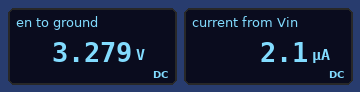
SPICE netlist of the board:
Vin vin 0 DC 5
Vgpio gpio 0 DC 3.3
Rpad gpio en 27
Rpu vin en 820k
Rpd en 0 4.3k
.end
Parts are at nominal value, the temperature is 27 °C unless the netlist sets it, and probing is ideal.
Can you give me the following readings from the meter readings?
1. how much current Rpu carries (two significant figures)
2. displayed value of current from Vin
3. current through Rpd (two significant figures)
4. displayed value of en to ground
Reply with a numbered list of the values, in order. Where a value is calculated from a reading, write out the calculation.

1. (5 V - 3.279 V) / 820 kΩ = 2.1 µA
2. 2.1 µA
3. (3.279 V) / 4.3 kΩ = 760 µA
4. 3.279 V
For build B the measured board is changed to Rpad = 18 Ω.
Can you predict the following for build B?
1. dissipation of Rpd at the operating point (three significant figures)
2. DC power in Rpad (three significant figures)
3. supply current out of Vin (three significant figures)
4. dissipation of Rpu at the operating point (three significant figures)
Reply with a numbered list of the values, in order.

1. 2.51 mW
2. 10.5 µW
3. 2.09 µA
4. 3.58 µW
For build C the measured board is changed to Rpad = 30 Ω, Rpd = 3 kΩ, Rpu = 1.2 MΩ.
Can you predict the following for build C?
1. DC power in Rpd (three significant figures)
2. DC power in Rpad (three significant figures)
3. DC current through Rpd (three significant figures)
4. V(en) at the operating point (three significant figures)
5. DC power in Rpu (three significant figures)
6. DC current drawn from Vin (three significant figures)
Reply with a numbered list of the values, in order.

1. 3.56 mW
2. 35.5 µW
3. 1.09 mA
4. 3.27 V
5. 2.50 µW
6. 1.44 µA
